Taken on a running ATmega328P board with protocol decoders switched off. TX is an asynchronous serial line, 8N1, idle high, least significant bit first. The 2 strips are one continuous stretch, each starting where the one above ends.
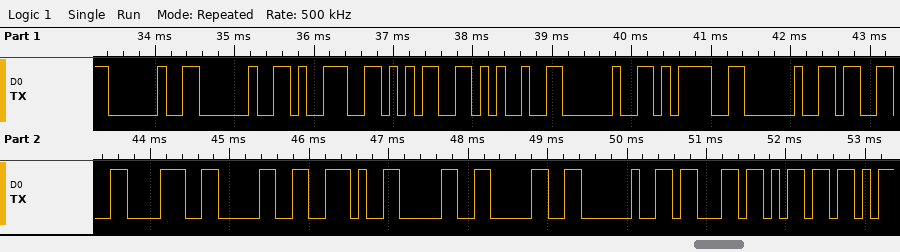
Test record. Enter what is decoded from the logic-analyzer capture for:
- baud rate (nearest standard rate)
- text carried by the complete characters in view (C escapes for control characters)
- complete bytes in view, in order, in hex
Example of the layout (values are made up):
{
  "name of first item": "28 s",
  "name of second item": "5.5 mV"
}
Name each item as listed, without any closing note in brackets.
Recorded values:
{
  "baud rate": "9600 baud",
  "text carried by the complete characters in view": "\"  95% = 380.00 cm\"",
  "complete bytes in view, in order, in hex": "0x20 0x20 0x39 0x35 0x25 0x20 0x3D 0x20 0x33 0x38 0x30 0x2E 0x30 0x30 0x20 0x63 0x6D"
}
